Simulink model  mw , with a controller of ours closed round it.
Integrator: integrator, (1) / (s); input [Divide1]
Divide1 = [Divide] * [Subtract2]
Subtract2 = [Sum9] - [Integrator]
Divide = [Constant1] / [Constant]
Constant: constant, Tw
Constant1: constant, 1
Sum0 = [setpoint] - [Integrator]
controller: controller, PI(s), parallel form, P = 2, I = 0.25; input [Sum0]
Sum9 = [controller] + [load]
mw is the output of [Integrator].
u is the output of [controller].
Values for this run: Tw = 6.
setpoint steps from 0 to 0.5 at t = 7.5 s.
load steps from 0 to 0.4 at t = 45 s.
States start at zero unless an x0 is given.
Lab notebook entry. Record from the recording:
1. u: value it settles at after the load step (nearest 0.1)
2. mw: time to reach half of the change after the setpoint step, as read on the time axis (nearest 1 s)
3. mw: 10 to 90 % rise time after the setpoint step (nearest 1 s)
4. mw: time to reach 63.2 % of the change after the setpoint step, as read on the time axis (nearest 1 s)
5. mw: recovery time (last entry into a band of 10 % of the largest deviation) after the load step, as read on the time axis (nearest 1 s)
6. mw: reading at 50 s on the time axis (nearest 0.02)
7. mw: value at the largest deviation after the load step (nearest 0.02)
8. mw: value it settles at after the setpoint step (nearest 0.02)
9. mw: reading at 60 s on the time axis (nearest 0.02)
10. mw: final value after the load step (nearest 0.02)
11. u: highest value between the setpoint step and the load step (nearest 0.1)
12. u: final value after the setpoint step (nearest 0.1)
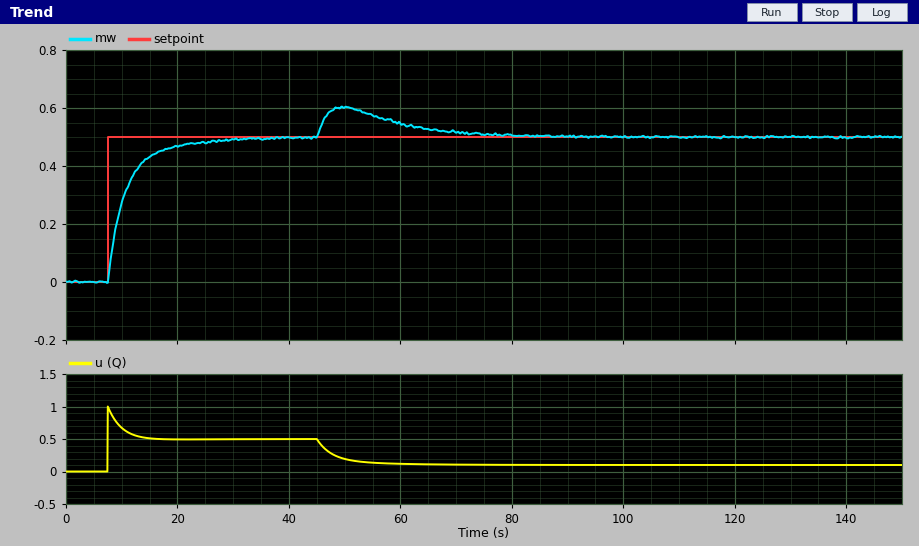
0.1
10 s
9 s
11 s
74 s
0.60
0.60
0.50
0.54
0.50
1.0
0.5
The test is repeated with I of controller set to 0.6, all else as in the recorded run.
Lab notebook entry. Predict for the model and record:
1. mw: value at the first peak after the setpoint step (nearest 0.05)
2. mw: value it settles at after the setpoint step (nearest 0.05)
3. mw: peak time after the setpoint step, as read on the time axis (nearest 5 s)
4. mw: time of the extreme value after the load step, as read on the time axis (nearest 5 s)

0.55
0.50
15 s
50 s
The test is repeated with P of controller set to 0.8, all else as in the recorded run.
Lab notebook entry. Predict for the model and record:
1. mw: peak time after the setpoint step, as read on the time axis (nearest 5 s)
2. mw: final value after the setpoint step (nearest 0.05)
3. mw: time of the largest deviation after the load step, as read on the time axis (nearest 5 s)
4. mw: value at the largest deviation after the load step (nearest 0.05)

25 s
0.50
50 s
0.65
